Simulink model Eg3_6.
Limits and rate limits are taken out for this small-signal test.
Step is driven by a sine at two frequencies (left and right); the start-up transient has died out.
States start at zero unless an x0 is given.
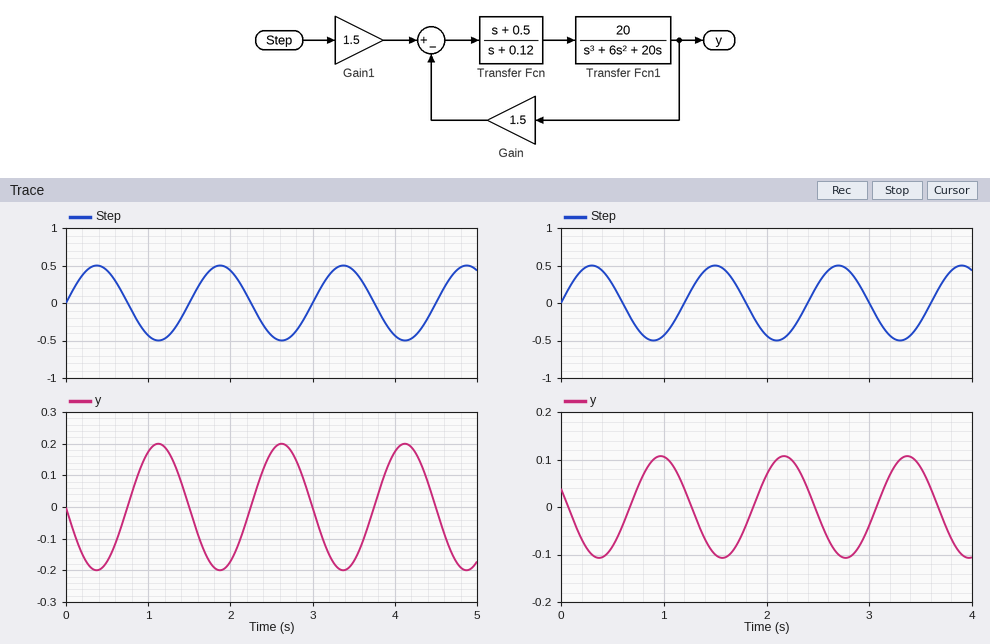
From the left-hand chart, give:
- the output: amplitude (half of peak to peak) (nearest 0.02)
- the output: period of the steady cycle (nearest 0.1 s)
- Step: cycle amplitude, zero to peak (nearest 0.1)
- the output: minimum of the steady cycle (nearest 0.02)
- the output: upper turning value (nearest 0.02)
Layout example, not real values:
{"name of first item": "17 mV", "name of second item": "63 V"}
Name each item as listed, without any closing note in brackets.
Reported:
{"the output: amplitude (half of peak to peak)": "0.20", "the output: period of the steady cycle": "1.5 s", "Step: cycle amplitude, zero to peak": "0.5", "the output: minimum of the steady cycle": "-0.20", "the output: upper turning value": "0.20"}
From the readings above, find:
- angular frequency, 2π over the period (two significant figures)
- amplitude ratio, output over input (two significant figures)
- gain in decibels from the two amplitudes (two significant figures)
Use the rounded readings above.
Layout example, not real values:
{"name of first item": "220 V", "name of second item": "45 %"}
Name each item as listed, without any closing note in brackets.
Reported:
{"angular frequency, 2π over the period": "4.2 rad/s", "amplitude ratio, output over input": "0.40", "gain in decibels from the two amplitudes": "-8.0 dB"}
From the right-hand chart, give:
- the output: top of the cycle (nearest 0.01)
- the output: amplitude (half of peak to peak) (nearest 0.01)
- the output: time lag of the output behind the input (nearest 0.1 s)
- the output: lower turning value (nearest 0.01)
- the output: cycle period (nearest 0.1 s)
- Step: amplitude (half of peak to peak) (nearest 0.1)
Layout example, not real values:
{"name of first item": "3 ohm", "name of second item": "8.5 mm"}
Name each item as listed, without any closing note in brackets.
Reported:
{"the output: top of the cycle": "0.11", "the output: amplitude (half of peak to peak)": "0.11", "the output: time lag of the output behind the input": "0.7 s", "the output: lower turning value": "-0.11", "the output: cycle period": "1.2 s", "Step: amplitude (half of peak to peak)": "0.5"}
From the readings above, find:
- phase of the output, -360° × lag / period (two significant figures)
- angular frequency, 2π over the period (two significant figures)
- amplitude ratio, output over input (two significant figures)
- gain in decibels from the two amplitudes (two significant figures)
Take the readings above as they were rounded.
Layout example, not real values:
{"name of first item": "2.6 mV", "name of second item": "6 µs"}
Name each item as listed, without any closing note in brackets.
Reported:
{"phase of the output, -360° × lag / period": "-210°", "angular frequency, 2π over the period": "5.2 rad/s", "amplitude ratio, output over input": "0.22", "gain in decibels from the two amplitudes": "-13 dB"}
